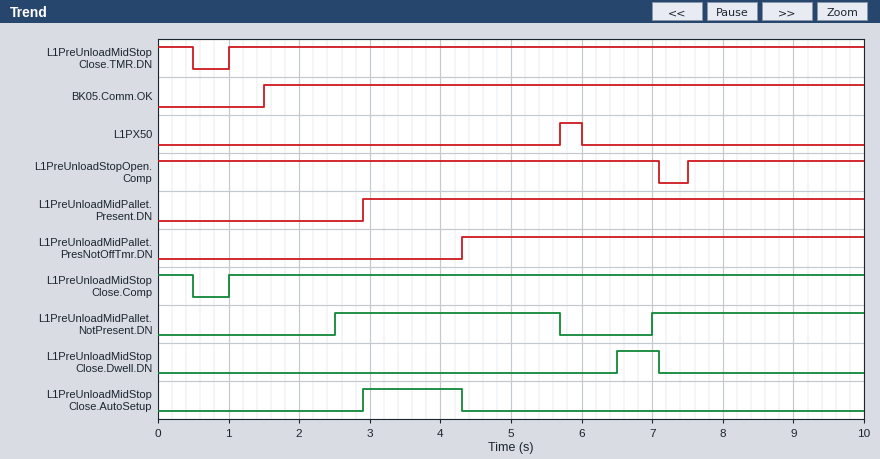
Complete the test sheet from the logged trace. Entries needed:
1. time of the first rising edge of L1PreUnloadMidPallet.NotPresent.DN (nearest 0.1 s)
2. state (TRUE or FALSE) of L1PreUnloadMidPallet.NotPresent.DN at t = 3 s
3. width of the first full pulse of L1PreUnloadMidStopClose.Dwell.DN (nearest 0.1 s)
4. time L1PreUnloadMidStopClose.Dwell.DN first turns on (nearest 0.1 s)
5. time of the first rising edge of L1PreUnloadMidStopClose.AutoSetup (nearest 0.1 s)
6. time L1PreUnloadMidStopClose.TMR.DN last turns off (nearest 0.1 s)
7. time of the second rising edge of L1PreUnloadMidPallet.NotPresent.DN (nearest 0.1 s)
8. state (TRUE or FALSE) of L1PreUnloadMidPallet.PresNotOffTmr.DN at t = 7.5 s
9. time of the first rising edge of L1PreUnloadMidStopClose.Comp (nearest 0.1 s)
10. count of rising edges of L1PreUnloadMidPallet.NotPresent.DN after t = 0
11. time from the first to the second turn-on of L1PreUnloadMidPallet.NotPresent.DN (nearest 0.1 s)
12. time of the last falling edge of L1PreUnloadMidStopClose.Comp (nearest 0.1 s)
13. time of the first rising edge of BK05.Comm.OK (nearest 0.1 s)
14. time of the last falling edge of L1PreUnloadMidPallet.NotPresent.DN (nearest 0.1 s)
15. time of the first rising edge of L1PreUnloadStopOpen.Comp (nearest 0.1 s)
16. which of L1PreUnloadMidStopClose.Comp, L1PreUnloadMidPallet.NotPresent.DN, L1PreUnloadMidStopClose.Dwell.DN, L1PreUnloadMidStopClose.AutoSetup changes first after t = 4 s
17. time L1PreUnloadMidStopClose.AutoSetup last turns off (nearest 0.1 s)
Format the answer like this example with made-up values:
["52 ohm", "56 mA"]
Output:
["2.5 s", "TRUE", "0.6 s", "6.5 s", "2.9 s", "0.5 s", "7.0 s", "TRUE", "1.0 s", "2", "4.5 s", "0.5 s", "1.5 s", "5.7 s", "7.5 s", "L1PreUnloadMidStopClose.AutoSetup", "4.3 s"]
